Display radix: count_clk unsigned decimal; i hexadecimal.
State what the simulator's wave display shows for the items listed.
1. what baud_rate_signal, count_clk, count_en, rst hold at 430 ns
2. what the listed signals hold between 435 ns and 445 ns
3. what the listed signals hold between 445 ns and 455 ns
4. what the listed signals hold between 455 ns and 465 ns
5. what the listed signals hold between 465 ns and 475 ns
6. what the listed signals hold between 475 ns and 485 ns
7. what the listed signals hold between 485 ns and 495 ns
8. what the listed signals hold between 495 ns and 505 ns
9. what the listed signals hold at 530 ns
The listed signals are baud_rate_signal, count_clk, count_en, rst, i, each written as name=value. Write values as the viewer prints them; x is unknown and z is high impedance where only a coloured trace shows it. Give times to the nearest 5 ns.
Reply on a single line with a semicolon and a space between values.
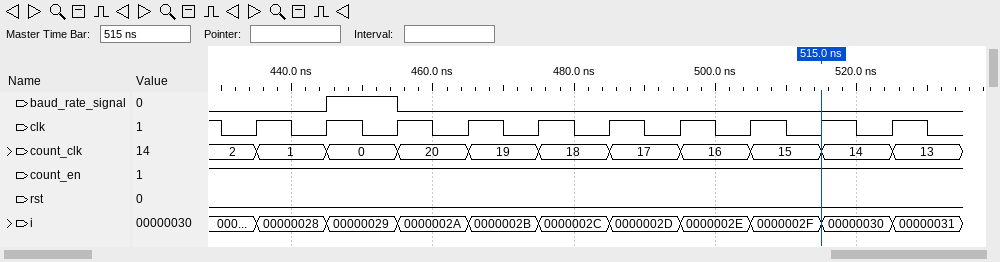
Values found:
baud_rate_signal=0, count_clk=2, count_en=1, rst=0; baud_rate_signal=0, count_clk=1, count_en=1, rst=0, i=00000028; baud_rate_signal=1, count_clk=0, count_en=1, rst=0, i=00000029; baud_rate_signal=0, count_clk=20, count_en=1, rst=0, i=0000002A; baud_rate_signal=0, count_clk=19, count_en=1, rst=0, i=0000002B; baud_rate_signal=0, count_clk=18, count_en=1, rst=0, i=0000002C; baud_rate_signal=0, count_clk=17, count_en=1, rst=0, i=0000002D; baud_rate_signal=0, count_clk=16, count_en=1, rst=0, i=0000002E; baud_rate_signal=0, count_clk=13, count_en=1, rst=0, i=00000031
